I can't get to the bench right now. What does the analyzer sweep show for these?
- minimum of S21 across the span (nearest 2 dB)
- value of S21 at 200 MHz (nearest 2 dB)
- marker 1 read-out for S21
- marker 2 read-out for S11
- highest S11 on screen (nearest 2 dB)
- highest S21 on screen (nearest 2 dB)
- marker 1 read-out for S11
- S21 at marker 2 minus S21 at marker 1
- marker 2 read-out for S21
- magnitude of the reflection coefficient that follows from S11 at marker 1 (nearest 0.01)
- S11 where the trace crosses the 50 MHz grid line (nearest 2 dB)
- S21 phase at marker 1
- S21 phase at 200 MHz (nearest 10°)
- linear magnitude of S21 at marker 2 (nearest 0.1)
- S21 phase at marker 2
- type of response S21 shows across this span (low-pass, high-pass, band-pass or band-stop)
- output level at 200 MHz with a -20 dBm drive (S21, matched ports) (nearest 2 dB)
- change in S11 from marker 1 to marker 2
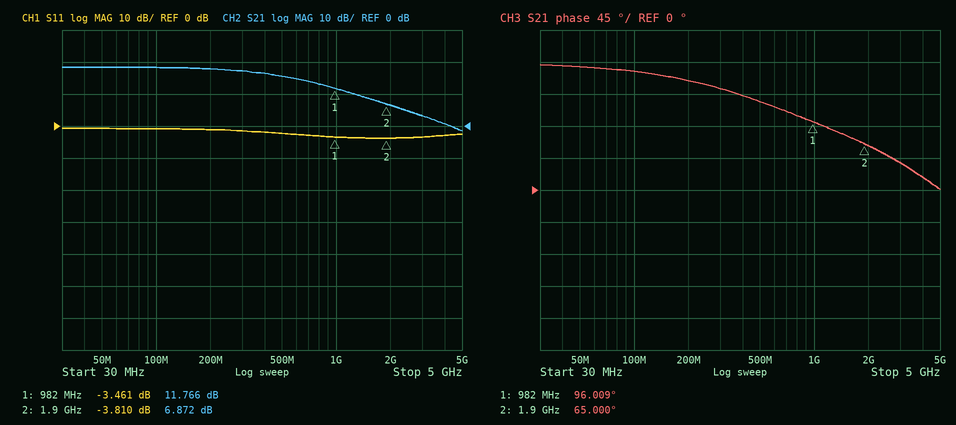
-2 dB
18 dB
11.766 dB
-3.810 dB
0 dB
18 dB
-3.461 dB
-4.894 dB
6.872 dB
0.67
0 dB
96.009°
150°
2.2
65.000°
low-pass
-2 dBm
-0.349 dB
